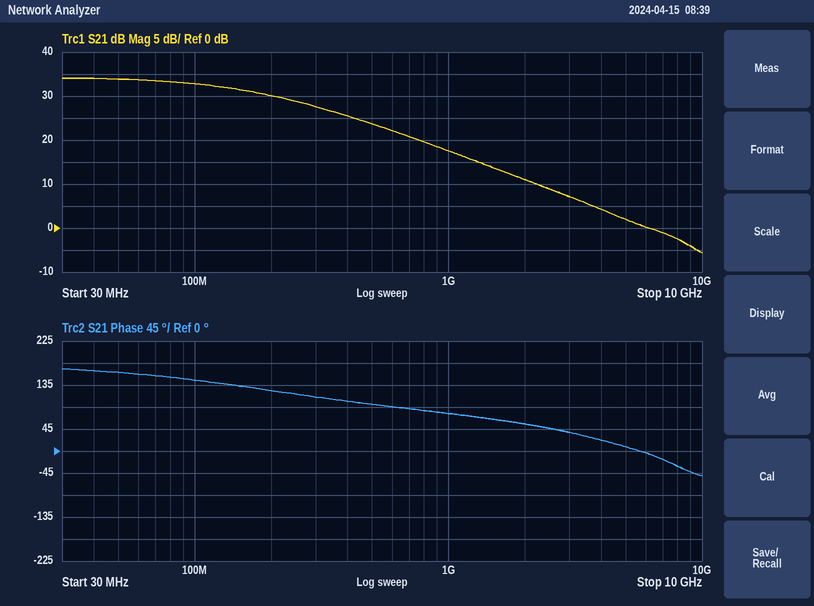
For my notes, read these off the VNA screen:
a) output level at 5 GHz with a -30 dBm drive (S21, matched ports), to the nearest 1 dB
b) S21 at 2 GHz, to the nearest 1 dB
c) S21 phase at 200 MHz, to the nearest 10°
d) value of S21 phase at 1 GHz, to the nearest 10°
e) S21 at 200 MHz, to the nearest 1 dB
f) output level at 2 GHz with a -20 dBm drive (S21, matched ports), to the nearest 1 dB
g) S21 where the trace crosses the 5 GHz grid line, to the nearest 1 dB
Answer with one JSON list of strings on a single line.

["-28 dBm", "11 dB", "120°", "80°", "30 dB", "-9 dBm", "2 dB"]
